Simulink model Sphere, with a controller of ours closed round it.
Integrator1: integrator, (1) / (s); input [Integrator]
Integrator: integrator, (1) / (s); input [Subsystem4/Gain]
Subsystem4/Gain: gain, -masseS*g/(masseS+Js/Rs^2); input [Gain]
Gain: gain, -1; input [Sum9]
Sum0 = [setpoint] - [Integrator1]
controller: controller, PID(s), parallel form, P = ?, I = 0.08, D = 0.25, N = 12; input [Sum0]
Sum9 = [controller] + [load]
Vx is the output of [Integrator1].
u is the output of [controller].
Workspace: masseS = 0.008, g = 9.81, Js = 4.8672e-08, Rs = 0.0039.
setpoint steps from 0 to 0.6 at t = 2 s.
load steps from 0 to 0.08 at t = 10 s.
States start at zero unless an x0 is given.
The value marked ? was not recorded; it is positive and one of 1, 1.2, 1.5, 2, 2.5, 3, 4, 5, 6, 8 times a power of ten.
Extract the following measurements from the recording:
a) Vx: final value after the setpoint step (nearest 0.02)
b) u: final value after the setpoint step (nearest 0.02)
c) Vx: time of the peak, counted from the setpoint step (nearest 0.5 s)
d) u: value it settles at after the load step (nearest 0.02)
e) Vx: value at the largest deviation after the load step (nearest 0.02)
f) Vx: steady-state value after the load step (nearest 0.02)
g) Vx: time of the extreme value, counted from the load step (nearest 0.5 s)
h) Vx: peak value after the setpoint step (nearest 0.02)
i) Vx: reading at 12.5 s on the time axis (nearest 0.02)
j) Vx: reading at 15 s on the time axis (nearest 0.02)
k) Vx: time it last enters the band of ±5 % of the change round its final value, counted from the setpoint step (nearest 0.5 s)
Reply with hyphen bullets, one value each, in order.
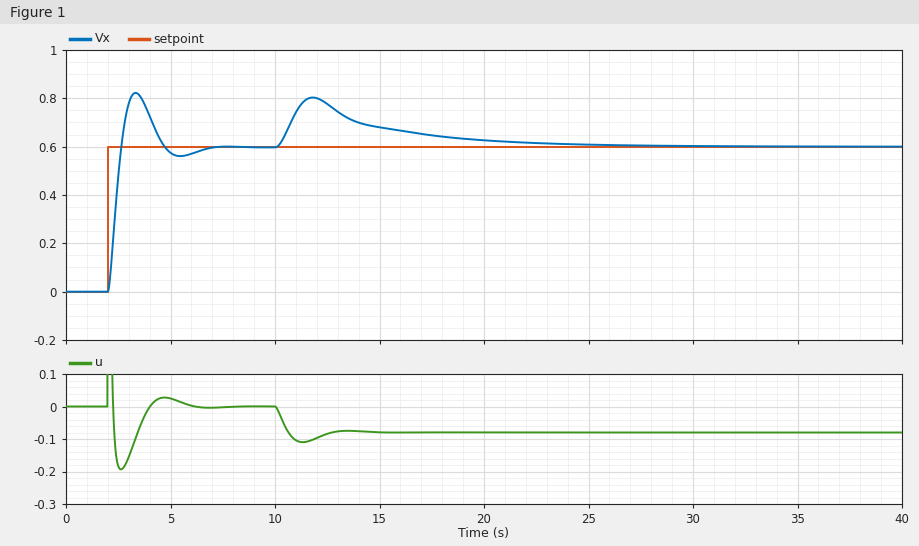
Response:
- 0.60
- 0.00
- 1.5 s
- -0.08
- 0.80
- 0.60
- 2.0 s
- 0.82
- 0.78
- 0.68
- 4.0 s
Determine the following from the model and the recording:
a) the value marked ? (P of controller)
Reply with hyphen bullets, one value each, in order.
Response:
- 0.4
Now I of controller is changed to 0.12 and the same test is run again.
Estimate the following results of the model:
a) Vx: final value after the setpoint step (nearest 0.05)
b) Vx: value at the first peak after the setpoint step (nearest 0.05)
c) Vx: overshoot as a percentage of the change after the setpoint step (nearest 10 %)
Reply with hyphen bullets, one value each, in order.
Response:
- 0.60
- 0.85
- 40 %
